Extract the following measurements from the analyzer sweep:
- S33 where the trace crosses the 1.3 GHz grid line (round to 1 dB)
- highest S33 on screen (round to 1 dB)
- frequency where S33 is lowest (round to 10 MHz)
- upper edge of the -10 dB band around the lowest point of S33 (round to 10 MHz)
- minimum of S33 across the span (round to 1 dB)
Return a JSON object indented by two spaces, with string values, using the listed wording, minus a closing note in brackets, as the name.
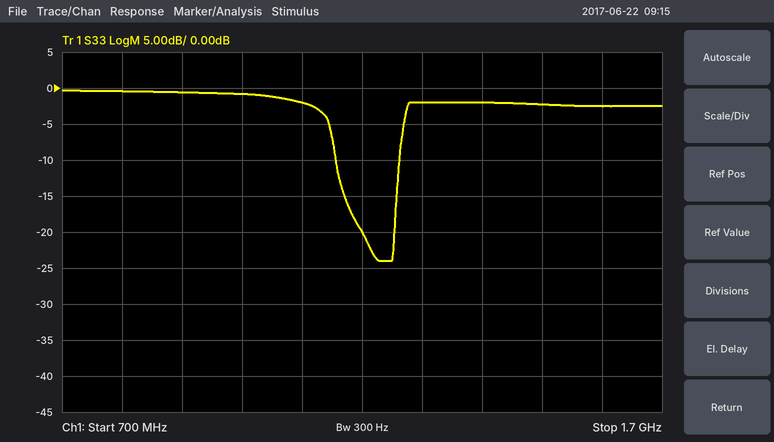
{
  "S33 where the trace crosses the 1.3 GHz grid line": "-2 dB",
  "highest S33 on screen": "0 dB",
  "frequency where S33 is lowest": "1.23 GHz",
  "upper edge of the -10 dB band around the lowest point of S33": "1.26 GHz",
  "minimum of S33 across the span": "-24 dB"
}
